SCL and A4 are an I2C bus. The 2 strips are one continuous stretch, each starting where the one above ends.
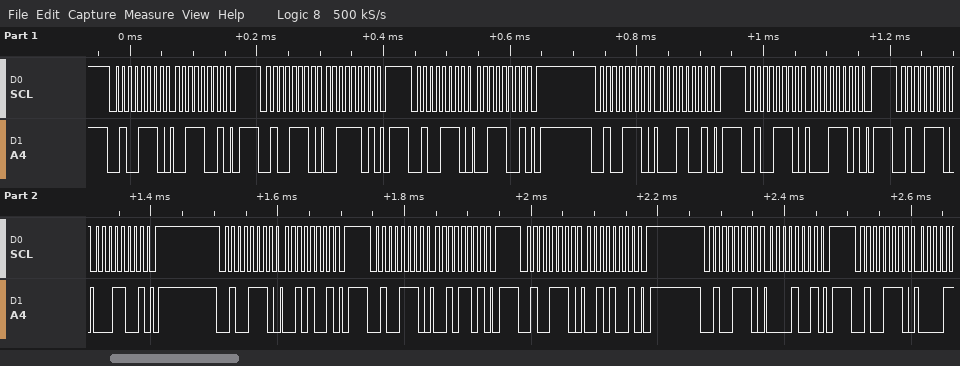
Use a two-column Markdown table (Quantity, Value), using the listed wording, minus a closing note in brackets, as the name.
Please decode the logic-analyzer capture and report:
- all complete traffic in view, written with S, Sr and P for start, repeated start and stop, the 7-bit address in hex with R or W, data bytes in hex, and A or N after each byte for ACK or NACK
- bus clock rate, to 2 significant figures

| Quantity | Value |
|---|---|
| all complete traffic in view, written with S, Sr and P for start, repeated start and stop, the 7-bit address in hex with R or W, data bytes in hex, and A or N after each byte for ACK or NACK | S 27W A 39 A P S 27W A 3D A P S 27W A 39 A P S 27W A 19 A P S 27W A 1D A P S 27W A 19 A P S 27W A 29 A P S 27W A 2D A P S 27W A 29 A P S 27W A 09 A P S 27W A |
| bus clock rate, to 2 significant figures | 100 kHz |
